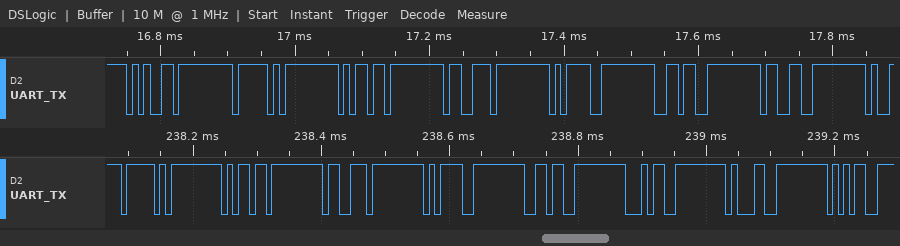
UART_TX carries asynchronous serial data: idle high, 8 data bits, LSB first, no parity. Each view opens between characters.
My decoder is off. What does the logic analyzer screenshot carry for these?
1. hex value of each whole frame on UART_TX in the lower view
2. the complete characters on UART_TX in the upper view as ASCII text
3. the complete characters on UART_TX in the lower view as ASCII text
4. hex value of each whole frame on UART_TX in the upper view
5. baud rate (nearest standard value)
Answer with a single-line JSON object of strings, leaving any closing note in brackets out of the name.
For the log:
{"hex value of each whole frame on UART_TX in the lower view": "5F, 6D, 73, 3D, 36, 34, 31, 35", "the complete characters on UART_TX in the upper view as ASCII text": "\"e_ms=63\"", "the complete characters on UART_TX in the lower view as ASCII text": "\"_ms=6415\"", "hex value of each whole frame on UART_TX in the upper view": "65, 5F, 6D, 73, 3D, 36, 33", "baud rate": "115200 baud"}
